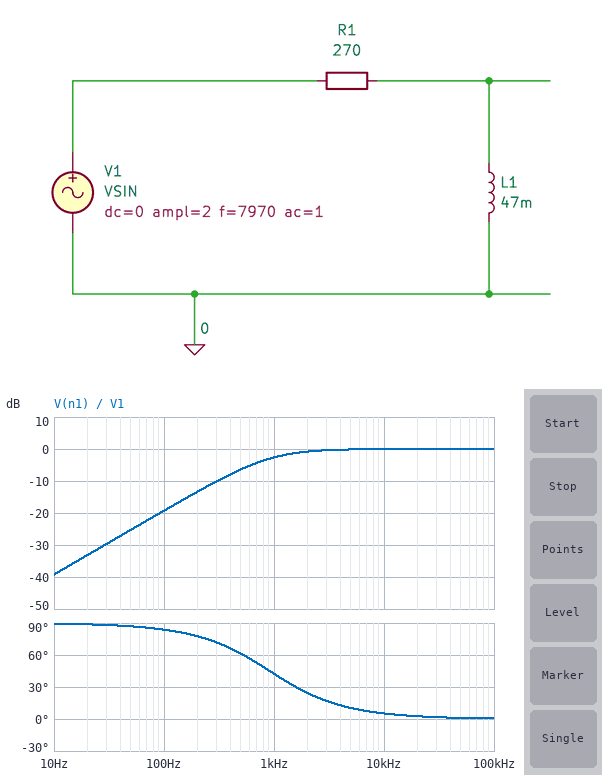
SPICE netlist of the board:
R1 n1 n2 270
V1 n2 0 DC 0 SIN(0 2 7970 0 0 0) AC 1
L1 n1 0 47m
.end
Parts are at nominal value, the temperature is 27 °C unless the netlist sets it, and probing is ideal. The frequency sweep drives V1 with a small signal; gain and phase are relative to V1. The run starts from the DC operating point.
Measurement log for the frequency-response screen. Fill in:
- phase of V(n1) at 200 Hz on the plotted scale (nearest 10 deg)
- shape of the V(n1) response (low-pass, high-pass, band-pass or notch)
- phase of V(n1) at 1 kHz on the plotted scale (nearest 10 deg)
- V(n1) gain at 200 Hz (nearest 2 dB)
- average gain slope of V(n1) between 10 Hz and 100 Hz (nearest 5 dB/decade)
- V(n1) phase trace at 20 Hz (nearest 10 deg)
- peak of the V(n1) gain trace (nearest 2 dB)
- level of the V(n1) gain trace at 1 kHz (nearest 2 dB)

80 deg
high-pass
40 deg
-14 dB
20 dB/decade
90 deg
0 dB
-2 dB
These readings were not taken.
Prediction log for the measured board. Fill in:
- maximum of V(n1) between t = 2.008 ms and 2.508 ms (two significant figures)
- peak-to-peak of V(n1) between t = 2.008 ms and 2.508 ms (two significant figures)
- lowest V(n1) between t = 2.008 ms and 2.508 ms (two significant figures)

2.0 V
4.0 V
-2.0 V
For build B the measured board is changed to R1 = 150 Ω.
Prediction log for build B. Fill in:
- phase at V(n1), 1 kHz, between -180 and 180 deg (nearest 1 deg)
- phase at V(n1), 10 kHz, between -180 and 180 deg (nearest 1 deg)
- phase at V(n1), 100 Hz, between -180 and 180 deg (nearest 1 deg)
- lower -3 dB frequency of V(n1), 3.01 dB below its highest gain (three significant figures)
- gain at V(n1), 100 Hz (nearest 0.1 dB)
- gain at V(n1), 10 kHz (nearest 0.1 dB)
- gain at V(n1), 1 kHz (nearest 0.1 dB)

27 deg
3 deg
79 deg
508 Hz
-14.3 dB
0 dB
-1.0 dB
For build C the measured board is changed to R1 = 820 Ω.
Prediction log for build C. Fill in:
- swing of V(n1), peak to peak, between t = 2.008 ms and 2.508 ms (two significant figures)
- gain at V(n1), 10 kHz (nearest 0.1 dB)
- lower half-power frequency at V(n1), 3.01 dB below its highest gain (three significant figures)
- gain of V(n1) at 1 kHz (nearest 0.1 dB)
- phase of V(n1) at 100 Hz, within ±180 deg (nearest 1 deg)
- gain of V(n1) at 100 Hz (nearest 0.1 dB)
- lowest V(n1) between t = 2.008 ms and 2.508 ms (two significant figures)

3.8 V
-0.3 dB
2.78 kHz
-9.4 dB
88 deg
-28.9 dB
-1.9 V
